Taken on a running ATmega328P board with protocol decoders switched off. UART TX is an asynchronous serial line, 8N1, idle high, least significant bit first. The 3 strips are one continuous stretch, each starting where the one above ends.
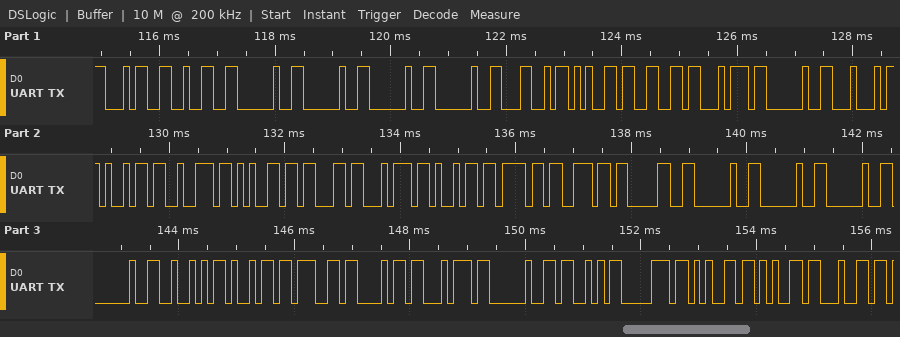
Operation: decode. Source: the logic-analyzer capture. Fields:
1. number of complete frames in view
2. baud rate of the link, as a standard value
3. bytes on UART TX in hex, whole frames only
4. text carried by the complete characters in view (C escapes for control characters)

36
9600 baud
34 32 20 20 20 20 4C 65 66 74 20 44 69 72 65 63 74 69 6F 6E 30 20 20 20 20 52 69 67 68 74 20 53 70 65 65 64
"42    Left Direction0    Right Speed"
